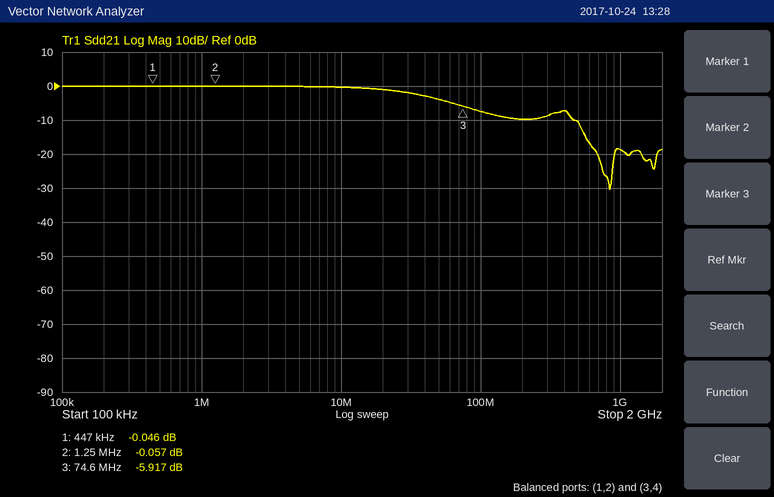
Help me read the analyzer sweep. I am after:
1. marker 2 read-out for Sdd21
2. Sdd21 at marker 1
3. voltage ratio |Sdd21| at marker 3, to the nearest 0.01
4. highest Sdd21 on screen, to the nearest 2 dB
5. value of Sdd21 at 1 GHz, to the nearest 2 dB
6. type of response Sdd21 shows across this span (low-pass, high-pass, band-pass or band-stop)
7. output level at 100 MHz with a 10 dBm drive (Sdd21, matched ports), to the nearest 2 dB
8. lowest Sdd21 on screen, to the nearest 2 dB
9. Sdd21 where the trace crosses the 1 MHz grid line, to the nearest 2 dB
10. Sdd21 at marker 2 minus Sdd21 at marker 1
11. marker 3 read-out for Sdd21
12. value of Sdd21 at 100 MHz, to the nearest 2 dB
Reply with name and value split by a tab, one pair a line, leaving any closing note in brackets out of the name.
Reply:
marker 2 read-out for Sdd21	-0.057 dB
Sdd21 at marker 1	-0.046 dB
voltage ratio |Sdd21| at marker 3, to the nearest 0.01	0.51
highest Sdd21 on screen, to the nearest 2 dB	0 dB
value of Sdd21 at 1 GHz, to the nearest 2 dB	-18 dB
type of response Sdd21 shows across this span	low-pass
output level at 100 MHz with a 10 dBm drive (Sdd21, matched ports), to the nearest 2 dB	2 dBm
lowest Sdd21 on screen, to the nearest 2 dB	-30 dB
Sdd21 where the trace crosses the 1 MHz grid line, to the nearest 2 dB	0 dB
Sdd21 at marker 2 minus Sdd21 at marker 1	-0.011 dB
marker 3 read-out for Sdd21	-5.917 dB
value of Sdd21 at 100 MHz, to the nearest 2 dB	-8 dB
